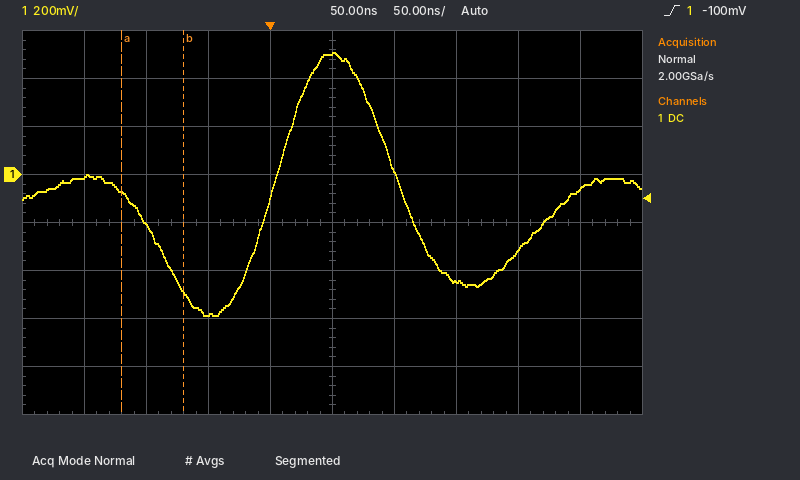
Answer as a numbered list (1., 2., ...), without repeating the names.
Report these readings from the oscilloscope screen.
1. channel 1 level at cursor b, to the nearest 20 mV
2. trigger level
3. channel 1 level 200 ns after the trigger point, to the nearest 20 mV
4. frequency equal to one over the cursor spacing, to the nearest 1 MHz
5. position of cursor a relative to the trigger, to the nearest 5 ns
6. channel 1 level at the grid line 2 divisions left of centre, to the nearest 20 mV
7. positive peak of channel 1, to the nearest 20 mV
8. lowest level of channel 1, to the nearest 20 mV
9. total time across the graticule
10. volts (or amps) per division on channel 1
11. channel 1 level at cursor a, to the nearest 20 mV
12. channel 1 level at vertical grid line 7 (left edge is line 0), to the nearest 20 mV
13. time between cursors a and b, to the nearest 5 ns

1. -480 mV
2. -100 mV
3. -320 mV
4. 20 MHz
5. -120 ns
6. -580 mV
7. 500 mV
8. -580 mV
9. 500 ns
10. 200 mV
11. -80 mV
12. -440 mV
13. 50 ns
